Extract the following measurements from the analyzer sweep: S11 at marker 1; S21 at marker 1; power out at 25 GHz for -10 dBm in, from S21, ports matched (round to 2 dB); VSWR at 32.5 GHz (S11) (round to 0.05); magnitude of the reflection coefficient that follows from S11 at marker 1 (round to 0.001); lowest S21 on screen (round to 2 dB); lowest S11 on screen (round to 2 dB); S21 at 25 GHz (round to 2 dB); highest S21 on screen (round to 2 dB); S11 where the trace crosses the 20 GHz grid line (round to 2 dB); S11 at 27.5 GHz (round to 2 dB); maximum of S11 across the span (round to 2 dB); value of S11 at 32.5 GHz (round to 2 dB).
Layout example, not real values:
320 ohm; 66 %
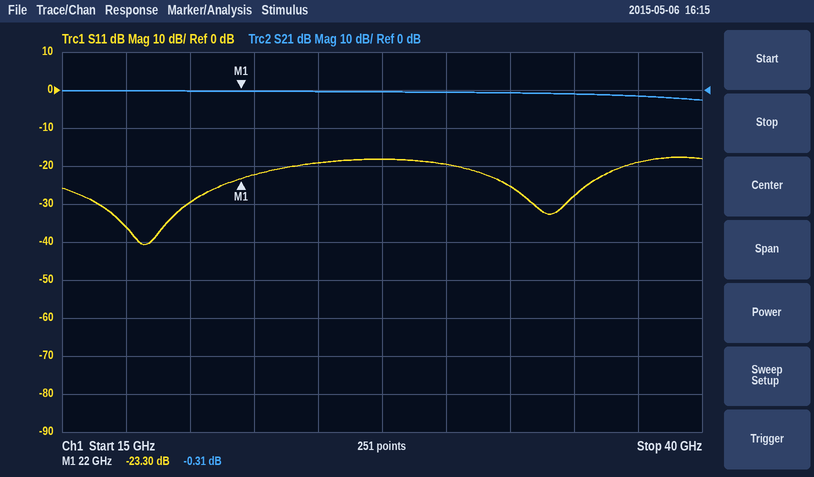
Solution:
-23.30 dB; -0.31 dB; -10 dBm; 1.10; 0.068; -2 dB; -40 dB; 0 dB; 0 dB; -30 dB; -18 dB; -18 dB; -26 dB
